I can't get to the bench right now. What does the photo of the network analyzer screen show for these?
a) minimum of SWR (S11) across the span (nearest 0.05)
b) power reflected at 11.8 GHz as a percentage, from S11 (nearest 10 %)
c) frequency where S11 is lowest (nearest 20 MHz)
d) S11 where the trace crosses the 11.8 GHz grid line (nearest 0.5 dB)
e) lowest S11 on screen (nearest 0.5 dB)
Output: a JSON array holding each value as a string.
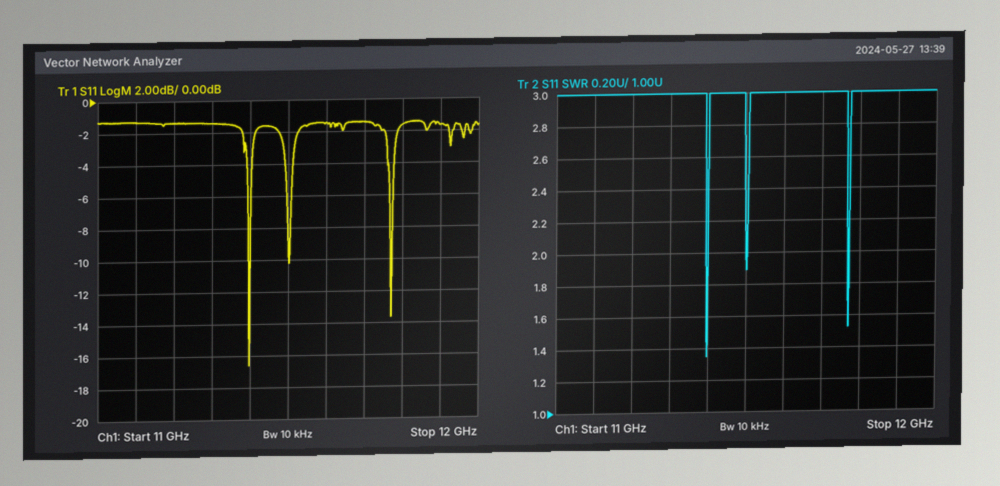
["1.35", "70 %", "11.40 GHz", "-1.5 dB", "-16.5 dB"]
